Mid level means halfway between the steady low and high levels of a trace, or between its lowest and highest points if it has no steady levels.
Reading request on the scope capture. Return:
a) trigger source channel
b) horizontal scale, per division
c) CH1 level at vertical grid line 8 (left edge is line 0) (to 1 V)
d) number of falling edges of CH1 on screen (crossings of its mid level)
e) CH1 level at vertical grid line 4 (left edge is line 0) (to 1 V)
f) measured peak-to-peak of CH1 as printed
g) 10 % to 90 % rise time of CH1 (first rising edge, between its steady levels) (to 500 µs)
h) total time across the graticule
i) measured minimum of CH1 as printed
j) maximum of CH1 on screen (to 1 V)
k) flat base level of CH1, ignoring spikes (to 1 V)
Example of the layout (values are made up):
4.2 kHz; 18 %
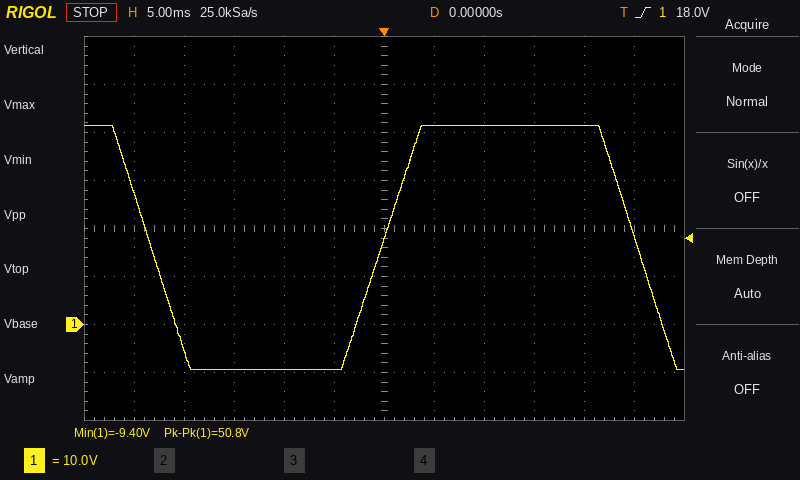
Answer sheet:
CH1; 5 ms; 41 V; 2; -9 V; 50.8 V; 6.5 ms; 60 ms; -9.40 V; 41 V; -9 V
